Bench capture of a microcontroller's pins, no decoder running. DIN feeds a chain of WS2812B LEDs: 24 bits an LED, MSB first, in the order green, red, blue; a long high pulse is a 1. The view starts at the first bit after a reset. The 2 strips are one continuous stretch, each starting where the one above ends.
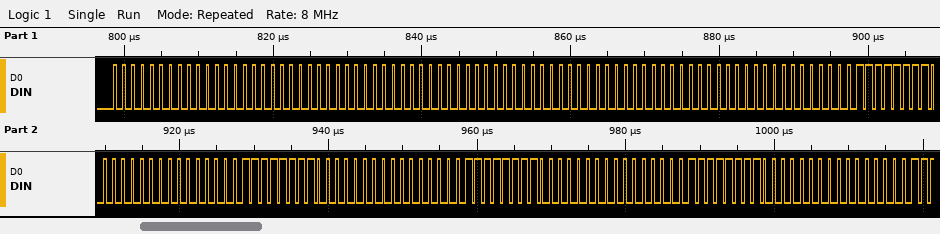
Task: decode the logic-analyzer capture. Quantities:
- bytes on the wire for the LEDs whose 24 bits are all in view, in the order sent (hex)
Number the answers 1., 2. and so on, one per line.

1. 00 00 00 00 00 00 00 00 00 00 FF 00 00 FF 00 00 FF 00 00 FF 00
